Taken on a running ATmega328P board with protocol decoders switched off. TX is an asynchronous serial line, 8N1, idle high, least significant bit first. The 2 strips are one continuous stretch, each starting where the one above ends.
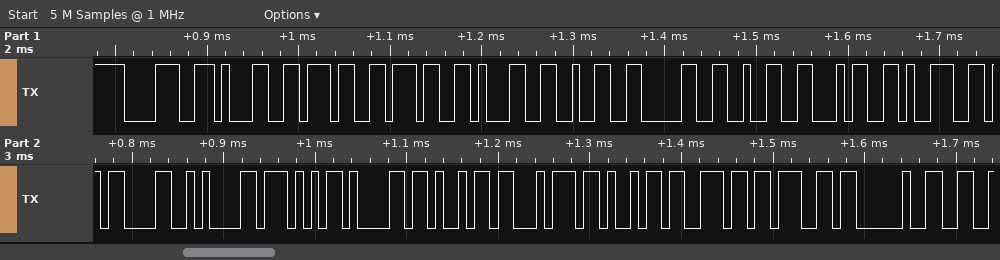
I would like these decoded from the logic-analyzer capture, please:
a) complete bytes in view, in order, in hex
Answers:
38 31 37 37 31 32 30 32 34 39 0D 0A 57 61 69 74 69 6E 67 20
